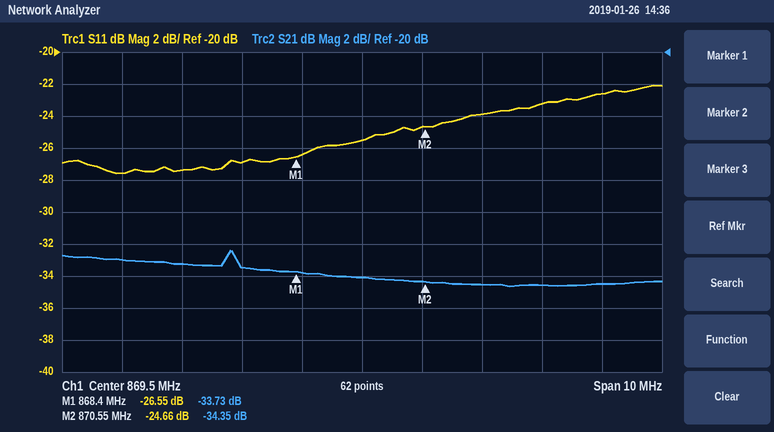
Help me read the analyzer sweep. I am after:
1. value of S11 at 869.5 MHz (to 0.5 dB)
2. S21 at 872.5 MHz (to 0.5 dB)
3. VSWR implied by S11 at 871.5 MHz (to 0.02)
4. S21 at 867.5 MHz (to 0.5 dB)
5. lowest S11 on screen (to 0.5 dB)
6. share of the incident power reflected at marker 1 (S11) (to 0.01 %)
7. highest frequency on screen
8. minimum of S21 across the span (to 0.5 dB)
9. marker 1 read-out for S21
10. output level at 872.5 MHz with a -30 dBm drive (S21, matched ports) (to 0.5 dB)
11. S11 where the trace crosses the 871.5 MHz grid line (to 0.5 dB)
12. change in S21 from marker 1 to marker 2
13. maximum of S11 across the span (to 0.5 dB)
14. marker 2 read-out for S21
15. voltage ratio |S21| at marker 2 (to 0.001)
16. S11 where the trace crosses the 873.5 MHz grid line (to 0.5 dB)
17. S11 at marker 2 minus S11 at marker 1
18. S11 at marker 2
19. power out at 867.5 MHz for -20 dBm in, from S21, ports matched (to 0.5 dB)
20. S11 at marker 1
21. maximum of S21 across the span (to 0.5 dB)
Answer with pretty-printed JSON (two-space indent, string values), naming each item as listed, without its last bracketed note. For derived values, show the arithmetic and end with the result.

{
  "value of S11 at 869.5 MHz": "-25.5 dB",
  "S21 at 872.5 MHz": "-34.5 dB",
  "VSWR implied by S11 at 871.5 MHz": "|Γ| = 10^(-24/20) = 0.0631; VSWR = (1 + 0.0631)/(1 − 0.0631) ≈ 1.13, so 1.14 to the nearest 0.02",
  "S21 at 867.5 MHz": "-33.5 dB",
  "lowest S11 on screen": "-27.5 dB",
  "share of the incident power reflected at marker 1 (S11)": "10^(-26.55/10) ≈ 0.22 %",
  "highest frequency on screen": "874.5 MHz",
  "minimum of S21 across the span": "-34.5 dB",
  "marker 1 read-out for S21": "-33.73 dB",
  "output level at 872.5 MHz with a -30 dBm drive (S21, matched ports)": "-30 dBm + (-34.5 dB) = -64.5 dBm",
  "S11 where the trace crosses the 871.5 MHz grid line": "-24.0 dB",
  "change in S21 from marker 1 to marker 2": "-34.35 − (-33.73) = -0.62 dB",
  "maximum of S11 across the span": "-22.0 dB",
  "marker 2 read-out for S21": "-34.35 dB",
  "voltage ratio |S21| at marker 2": "10^(-34.35/20) ≈ 0.019",
  "S11 where the trace crosses the 873.5 MHz grid line": "-22.5 dB",
  "S11 at marker 2 minus S11 at marker 1": "-24.66 − (-26.55) = 1.89 dB",
  "S11 at marker 2": "-24.66 dB",
  "power out at 867.5 MHz for -20 dBm in, from S21, ports matched": "-20 dBm + (-33.5 dB) = -53.5 dBm",
  "S11 at marker 1": "-26.55 dB",
  "maximum of S21 across the span": "-32.5 dB"
}
